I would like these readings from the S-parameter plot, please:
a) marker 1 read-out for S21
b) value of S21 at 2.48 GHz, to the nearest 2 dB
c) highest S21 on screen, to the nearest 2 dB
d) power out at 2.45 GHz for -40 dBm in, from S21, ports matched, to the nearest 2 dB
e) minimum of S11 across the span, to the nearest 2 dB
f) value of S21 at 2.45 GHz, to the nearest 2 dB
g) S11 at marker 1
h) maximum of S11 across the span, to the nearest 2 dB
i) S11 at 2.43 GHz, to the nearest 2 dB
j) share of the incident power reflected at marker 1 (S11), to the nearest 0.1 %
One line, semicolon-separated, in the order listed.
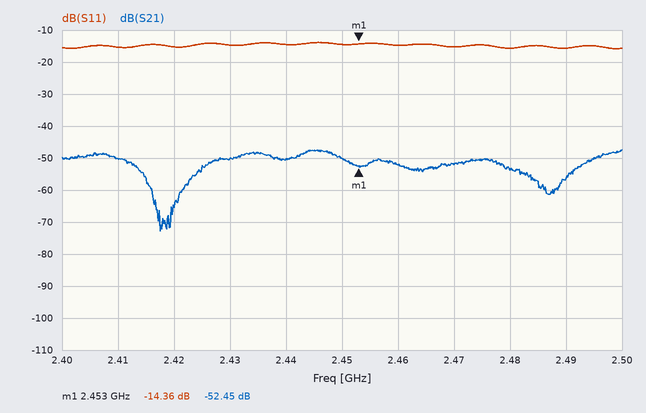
-52.45 dB; -54 dB; -48 dB; -90 dBm; -16 dB; -50 dB; -14.36 dB; -14 dB; -14 dB; 3.7 %
